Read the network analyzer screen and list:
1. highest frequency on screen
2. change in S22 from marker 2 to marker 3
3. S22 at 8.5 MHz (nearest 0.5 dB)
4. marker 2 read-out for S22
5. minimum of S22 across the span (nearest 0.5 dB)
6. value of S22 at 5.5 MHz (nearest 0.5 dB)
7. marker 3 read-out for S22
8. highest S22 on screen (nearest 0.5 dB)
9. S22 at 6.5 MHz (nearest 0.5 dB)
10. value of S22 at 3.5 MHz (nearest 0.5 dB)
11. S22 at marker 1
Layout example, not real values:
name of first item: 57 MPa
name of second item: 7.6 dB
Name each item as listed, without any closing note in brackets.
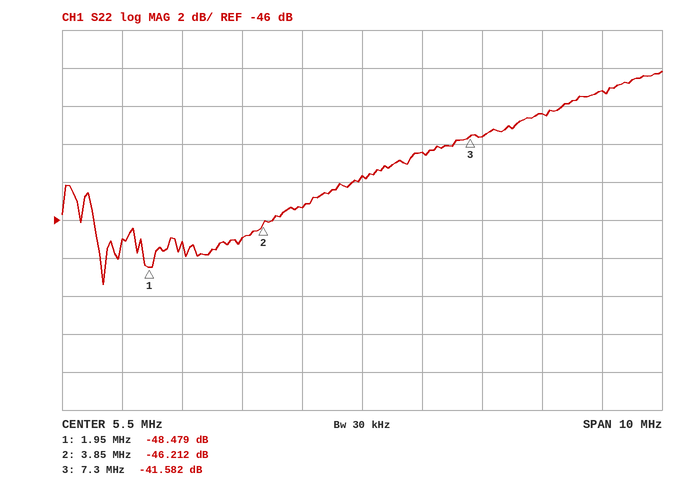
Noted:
highest frequency on screen: 10.5 MHz
change in S22 from marker 2 to marker 3: 4.630 dB
S22 at 8.5 MHz: -40.5 dB
marker 2 read-out for S22: -46.212 dB
minimum of S22 across the span: -49.5 dB
value of S22 at 5.5 MHz: -43.5 dB
marker 3 read-out for S22: -41.582 dB
highest S22 on screen: -38.0 dB
S22 at 6.5 MHz: -42.5 dB
value of S22 at 3.5 MHz: -47.0 dB
S22 at marker 1: -48.479 dB
